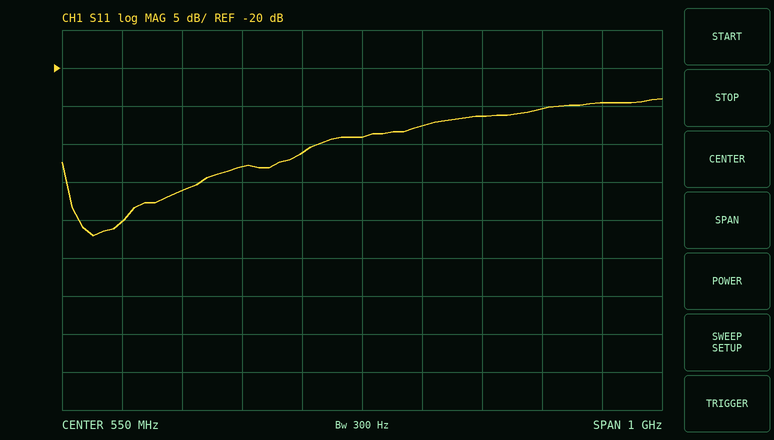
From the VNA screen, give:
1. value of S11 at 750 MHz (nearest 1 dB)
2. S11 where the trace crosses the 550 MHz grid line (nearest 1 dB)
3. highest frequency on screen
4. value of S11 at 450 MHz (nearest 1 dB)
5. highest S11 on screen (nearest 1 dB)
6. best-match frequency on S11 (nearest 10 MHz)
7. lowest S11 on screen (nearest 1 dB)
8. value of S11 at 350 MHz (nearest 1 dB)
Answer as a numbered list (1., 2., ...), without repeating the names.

1. -26 dB
2. -29 dB
3. 1.05 GHz
4. -31 dB
5. -24 dB
6. 100 MHz
7. -42 dB
8. -33 dB
